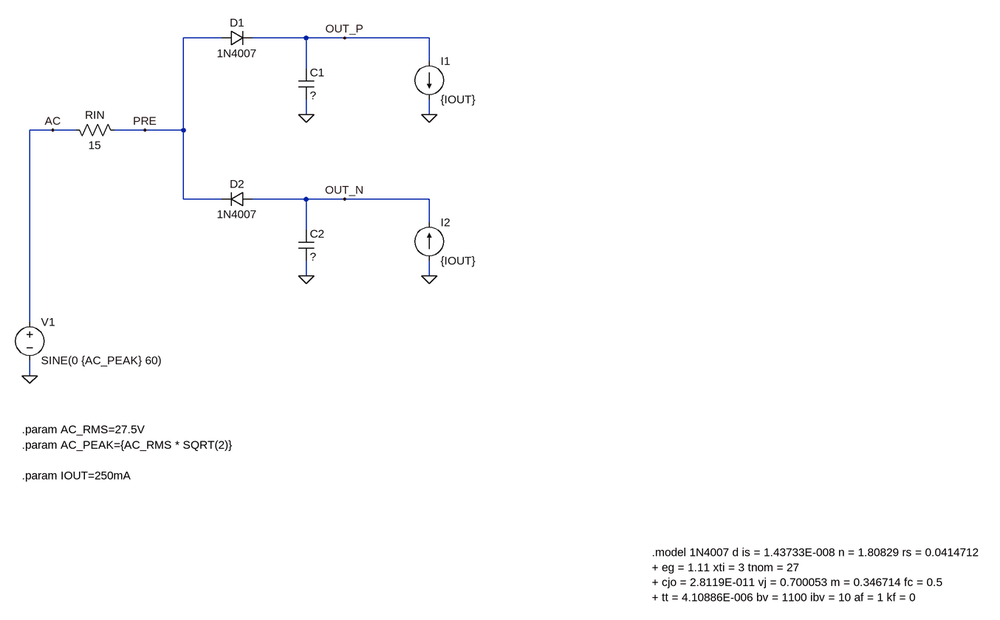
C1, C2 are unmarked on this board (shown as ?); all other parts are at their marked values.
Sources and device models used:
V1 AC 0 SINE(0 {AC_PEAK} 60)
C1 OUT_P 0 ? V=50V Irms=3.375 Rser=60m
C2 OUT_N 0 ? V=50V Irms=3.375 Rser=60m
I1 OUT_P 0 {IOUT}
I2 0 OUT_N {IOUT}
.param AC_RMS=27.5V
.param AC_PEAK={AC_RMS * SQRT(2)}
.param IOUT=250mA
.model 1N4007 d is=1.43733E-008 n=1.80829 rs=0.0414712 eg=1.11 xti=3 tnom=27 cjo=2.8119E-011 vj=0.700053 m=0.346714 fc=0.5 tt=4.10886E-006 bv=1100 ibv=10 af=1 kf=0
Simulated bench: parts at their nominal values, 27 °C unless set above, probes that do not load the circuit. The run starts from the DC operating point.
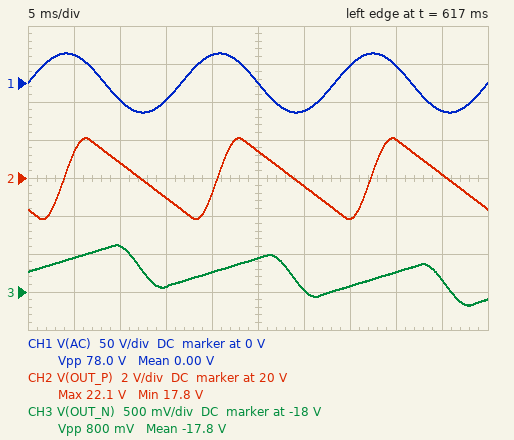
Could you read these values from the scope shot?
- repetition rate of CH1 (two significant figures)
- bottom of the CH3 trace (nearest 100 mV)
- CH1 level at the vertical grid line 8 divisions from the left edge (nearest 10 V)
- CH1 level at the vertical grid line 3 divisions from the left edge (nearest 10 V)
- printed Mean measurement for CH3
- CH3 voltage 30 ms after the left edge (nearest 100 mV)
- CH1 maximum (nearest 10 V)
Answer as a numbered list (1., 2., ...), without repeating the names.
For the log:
1. 60 Hz
2. -18.2 V
3. 20 V
4. -20 V
5. -17.8 V
6. -18.0 V
7. 40 V
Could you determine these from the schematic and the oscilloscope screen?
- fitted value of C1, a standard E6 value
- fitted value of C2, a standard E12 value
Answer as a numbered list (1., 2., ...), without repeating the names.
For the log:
1. 680 µF
2. 6.8 mF
